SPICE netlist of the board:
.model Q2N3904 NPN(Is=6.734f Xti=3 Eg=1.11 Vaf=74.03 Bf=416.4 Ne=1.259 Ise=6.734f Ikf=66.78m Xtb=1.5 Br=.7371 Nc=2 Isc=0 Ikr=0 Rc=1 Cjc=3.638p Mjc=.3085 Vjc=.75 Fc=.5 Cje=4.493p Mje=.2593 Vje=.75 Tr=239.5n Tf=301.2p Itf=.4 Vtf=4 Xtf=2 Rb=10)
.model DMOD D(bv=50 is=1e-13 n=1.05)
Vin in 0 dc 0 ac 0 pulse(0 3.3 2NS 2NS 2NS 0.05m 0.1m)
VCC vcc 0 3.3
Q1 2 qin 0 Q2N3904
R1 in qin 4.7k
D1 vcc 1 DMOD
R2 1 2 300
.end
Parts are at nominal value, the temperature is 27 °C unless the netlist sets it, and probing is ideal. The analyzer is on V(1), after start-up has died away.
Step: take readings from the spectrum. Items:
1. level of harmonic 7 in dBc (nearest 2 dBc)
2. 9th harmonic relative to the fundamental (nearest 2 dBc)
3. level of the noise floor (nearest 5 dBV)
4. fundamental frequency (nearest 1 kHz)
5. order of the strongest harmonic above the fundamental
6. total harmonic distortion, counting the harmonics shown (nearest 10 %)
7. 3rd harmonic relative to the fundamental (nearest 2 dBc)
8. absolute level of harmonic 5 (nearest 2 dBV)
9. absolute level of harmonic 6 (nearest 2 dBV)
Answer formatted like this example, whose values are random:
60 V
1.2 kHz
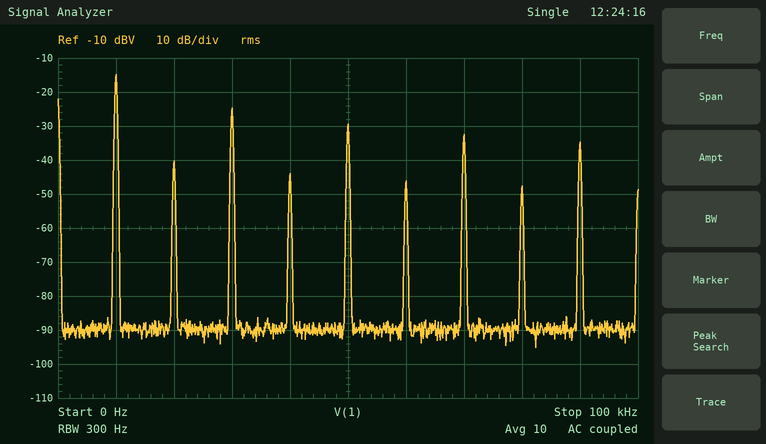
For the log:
-18 dBc
-20 dBc
-90 dBV
10 kHz
3
40 %
-10 dBc
-30 dBV
-46 dBV
